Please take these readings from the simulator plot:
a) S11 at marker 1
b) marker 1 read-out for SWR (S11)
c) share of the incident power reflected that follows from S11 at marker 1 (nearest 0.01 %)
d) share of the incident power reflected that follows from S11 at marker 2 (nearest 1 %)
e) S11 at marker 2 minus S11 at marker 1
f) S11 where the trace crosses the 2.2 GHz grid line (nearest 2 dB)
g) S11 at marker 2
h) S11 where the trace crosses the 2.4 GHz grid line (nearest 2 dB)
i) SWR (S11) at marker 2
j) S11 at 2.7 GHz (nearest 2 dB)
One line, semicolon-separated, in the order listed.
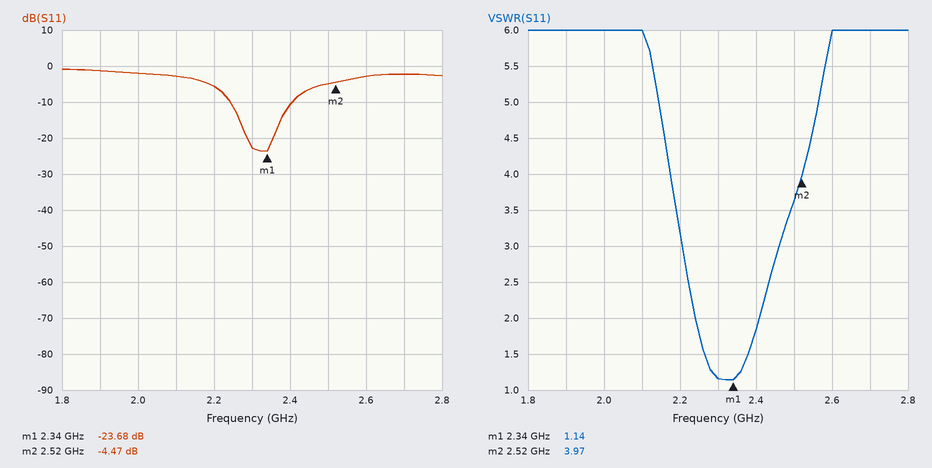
-23.68 dB; 1.14; 0.43 %; 36 %; 19.21 dB; -6 dB; -4.47 dB; -10 dB; 3.97; -2 dB
